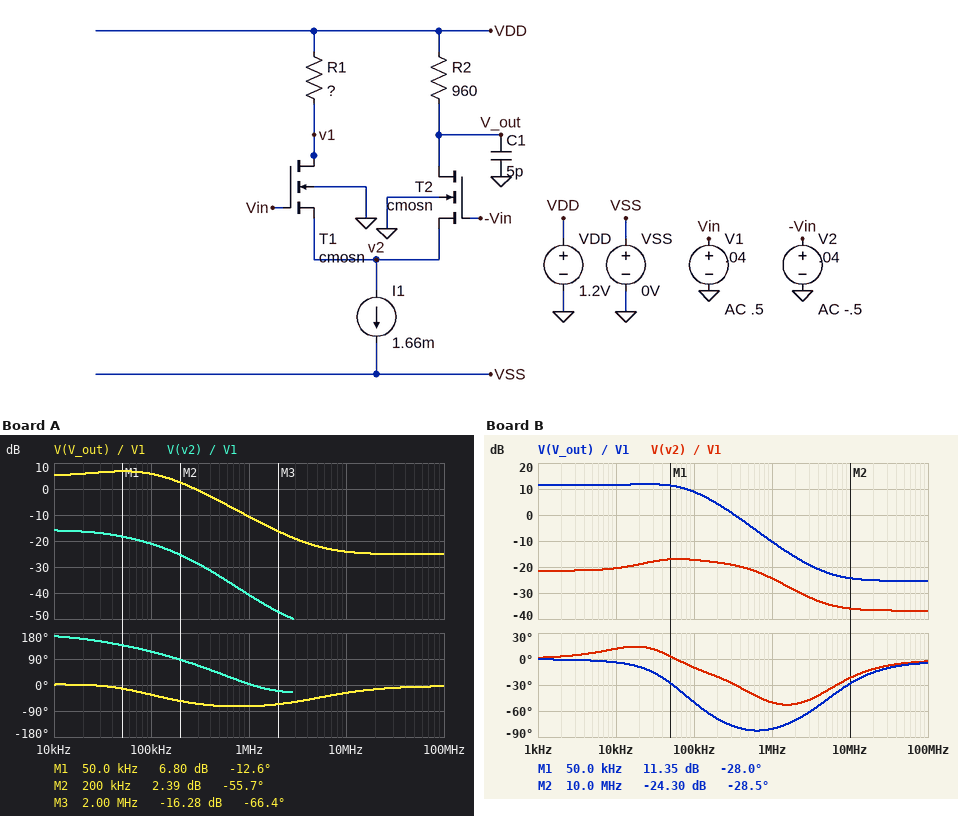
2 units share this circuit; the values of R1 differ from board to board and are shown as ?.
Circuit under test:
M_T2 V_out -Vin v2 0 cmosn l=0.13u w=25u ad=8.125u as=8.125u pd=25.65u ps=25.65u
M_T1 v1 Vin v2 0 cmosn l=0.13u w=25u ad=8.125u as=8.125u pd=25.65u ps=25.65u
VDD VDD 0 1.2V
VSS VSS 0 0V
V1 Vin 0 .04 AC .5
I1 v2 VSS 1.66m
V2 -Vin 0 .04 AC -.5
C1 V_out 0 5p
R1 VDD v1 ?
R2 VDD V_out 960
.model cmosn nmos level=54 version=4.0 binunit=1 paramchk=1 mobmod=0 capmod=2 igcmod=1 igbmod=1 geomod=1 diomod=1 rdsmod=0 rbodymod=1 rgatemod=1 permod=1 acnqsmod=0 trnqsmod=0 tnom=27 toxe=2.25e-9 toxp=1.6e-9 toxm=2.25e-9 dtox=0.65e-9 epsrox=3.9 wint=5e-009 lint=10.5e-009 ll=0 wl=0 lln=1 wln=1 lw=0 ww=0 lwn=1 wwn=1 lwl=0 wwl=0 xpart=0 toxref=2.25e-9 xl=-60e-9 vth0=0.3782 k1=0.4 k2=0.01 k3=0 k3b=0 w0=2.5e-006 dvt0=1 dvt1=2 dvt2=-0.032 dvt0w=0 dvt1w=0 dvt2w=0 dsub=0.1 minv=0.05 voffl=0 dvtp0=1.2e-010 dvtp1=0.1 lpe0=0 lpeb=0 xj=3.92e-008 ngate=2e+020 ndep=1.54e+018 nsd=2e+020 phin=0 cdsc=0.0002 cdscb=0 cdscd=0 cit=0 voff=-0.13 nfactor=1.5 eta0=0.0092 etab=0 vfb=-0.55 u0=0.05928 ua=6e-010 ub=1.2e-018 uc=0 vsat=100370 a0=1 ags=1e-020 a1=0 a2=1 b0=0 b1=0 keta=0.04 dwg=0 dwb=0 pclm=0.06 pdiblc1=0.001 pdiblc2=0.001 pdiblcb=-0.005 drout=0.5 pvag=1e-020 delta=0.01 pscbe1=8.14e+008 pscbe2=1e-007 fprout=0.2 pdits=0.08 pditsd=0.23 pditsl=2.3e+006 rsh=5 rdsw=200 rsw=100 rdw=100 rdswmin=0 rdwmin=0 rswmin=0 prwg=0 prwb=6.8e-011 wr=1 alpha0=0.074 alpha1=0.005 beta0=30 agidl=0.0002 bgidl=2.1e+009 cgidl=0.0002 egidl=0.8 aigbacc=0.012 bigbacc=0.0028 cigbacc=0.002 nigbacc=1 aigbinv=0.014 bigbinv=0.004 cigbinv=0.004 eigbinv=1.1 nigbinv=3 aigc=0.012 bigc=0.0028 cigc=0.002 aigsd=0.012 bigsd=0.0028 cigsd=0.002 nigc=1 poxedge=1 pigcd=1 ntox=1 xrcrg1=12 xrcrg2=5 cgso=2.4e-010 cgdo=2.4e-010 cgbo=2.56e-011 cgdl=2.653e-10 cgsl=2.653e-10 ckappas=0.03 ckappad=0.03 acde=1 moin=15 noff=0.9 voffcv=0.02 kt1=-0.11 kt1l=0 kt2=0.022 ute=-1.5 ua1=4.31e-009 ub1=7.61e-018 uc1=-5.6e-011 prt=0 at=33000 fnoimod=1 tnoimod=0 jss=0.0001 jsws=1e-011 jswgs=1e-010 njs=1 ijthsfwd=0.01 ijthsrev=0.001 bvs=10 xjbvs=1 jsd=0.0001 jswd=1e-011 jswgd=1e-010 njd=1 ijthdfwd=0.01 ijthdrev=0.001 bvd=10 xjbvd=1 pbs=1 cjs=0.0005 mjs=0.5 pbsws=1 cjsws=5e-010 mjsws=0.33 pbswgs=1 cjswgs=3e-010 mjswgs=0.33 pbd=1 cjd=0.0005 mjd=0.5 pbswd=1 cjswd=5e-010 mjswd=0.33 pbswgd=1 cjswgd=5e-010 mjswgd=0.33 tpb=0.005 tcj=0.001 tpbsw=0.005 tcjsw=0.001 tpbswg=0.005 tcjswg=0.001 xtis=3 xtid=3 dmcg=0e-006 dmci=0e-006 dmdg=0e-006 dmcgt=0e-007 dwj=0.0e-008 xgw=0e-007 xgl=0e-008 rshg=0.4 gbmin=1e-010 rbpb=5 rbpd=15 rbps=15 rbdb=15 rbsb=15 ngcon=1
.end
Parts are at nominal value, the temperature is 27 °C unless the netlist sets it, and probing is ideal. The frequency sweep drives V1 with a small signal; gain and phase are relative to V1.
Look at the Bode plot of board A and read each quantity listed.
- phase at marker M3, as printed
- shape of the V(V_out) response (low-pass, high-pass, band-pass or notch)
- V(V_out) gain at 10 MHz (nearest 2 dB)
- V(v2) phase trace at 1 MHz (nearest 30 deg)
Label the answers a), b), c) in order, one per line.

a) -66.4 deg
b) low-pass
c) -24 dB
d) 0 deg
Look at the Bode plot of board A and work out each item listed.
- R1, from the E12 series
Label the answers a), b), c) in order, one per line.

a) 2.7 kΩ
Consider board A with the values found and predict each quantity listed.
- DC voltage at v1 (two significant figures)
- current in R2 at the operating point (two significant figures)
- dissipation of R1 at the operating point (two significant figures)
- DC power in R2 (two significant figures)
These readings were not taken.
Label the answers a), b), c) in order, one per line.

a) -220 mV
b) 1.0 mA
c) 750 µW
d) 1.0 mW
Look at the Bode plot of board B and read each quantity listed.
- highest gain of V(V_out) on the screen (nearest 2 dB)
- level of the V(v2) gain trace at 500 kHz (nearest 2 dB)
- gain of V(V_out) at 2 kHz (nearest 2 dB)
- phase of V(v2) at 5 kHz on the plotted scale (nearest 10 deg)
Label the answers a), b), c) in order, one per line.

a) 12 dB
b) -20 dB
c) 12 dB
d) 10 deg
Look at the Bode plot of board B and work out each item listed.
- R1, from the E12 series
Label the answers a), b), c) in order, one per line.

a) 1.5 kΩ
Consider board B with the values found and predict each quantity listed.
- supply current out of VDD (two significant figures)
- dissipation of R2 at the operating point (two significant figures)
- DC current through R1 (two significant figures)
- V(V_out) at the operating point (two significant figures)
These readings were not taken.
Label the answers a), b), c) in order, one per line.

a) 1.6 mA
b) 770 µW
c) 710 µA
d) 340 mV
